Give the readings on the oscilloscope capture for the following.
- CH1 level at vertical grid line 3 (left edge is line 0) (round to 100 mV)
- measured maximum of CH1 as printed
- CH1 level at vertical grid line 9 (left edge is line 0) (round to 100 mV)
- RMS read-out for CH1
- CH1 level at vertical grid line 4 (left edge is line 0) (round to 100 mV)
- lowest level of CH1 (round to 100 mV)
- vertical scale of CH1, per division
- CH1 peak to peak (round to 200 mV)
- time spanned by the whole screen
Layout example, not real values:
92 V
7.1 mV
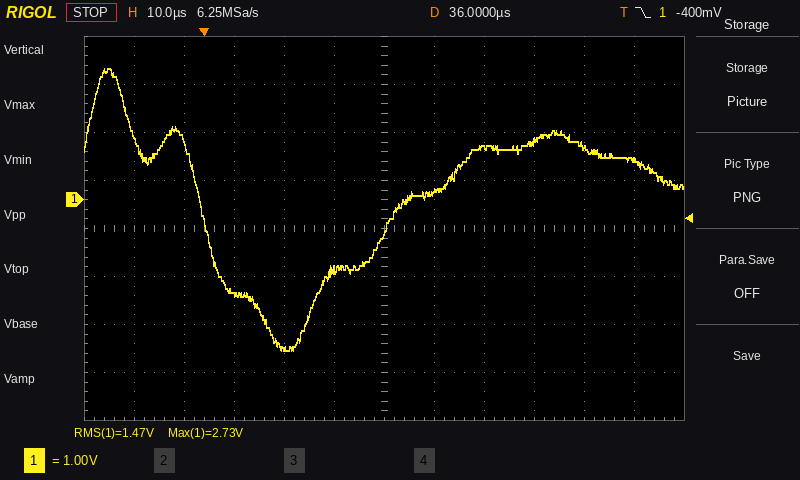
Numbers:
-2.0 V
2.73 V
1.2 V
1.47 V
-3.1 V
-3.1 V
1 V
5.8 V
120 µs
